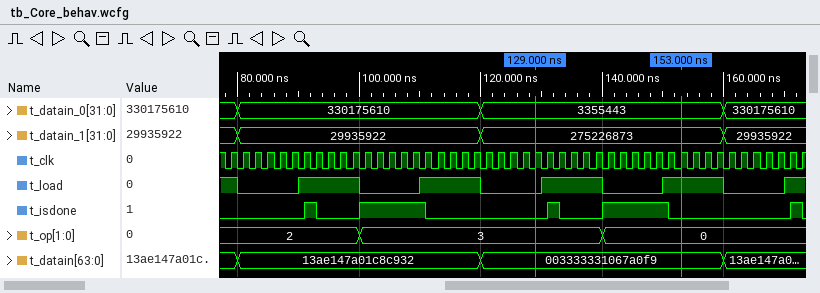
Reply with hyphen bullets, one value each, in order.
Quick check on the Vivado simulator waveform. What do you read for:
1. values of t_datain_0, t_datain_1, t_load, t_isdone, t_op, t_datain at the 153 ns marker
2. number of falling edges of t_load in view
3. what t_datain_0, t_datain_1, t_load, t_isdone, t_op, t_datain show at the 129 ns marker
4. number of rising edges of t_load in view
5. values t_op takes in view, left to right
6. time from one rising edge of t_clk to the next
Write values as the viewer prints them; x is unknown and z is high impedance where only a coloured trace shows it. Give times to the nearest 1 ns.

- t_datain_0=3355443, t_datain_1=275226873, t_load=1, t_isdone=0, t_op=0, t_datain=003333331067a0f9
- 5
- t_datain_0=3355443, t_datain_1=275226873, t_load=0, t_isdone=0, t_op=3, t_datain=003333331067a0f9
- 5
- 2, 3, 0
- 2 ns
